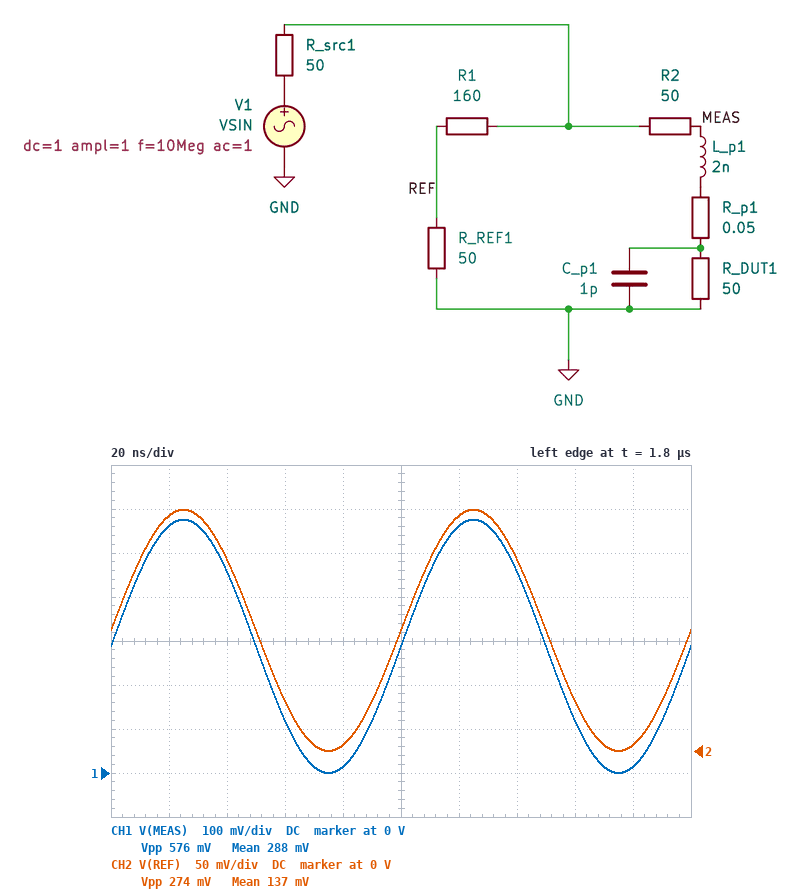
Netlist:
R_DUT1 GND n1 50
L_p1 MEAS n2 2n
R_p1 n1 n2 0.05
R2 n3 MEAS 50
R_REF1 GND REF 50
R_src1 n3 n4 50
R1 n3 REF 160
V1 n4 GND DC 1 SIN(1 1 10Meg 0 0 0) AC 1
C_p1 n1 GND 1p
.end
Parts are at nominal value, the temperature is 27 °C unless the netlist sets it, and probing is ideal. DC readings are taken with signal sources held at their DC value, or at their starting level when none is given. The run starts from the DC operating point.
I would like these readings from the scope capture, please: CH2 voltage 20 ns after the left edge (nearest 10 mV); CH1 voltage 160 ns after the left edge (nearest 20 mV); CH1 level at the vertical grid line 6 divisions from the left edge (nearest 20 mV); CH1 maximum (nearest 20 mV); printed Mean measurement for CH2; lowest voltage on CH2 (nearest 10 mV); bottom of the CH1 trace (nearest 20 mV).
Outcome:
270 mV
120 mV
560 mV
580 mV
137 mV
0 V
0 V
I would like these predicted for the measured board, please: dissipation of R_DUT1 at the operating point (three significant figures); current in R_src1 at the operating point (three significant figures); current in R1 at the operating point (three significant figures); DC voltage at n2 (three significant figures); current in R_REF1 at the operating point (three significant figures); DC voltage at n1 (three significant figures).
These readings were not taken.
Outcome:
1.65 mW
8.49 mA
2.74 mA
288 mV
2.74 mA
288 mV
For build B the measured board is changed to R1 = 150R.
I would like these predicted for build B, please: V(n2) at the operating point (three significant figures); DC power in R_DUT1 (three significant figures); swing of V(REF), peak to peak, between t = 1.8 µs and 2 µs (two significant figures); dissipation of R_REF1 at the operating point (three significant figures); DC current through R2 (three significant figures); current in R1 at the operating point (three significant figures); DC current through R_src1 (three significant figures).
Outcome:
286 mV
1.63 mW
290 mV
408 µW
5.71 mA
2.86 mA
8.57 mA
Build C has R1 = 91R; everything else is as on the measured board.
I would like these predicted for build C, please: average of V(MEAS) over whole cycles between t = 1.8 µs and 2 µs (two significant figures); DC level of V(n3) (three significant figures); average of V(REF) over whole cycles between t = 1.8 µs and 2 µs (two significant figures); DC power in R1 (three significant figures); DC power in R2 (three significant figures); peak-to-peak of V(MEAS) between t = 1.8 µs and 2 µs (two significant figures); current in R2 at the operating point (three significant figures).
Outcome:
270 mV
539 mV
190 mV
1.33 mW
1.45 mW
540 mV
5.39 mA
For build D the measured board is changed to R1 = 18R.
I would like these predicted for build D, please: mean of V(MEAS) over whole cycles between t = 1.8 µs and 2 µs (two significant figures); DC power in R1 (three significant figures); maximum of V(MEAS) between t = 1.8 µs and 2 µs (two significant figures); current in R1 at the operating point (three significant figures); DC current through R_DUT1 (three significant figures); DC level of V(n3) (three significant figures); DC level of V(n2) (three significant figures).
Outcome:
220 mV
779 µW
450 mV
6.58 mA
4.47 mA
447 mV
224 mV
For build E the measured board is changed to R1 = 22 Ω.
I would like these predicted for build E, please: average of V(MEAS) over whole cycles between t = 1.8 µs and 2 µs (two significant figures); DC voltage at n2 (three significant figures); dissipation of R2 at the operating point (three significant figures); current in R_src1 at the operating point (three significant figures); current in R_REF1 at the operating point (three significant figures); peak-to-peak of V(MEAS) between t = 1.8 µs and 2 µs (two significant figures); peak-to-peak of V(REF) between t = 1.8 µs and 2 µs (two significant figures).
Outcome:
230 mV
228 mV
1.04 mW
10.9 mA
6.33 mA
460 mV
630 mV
